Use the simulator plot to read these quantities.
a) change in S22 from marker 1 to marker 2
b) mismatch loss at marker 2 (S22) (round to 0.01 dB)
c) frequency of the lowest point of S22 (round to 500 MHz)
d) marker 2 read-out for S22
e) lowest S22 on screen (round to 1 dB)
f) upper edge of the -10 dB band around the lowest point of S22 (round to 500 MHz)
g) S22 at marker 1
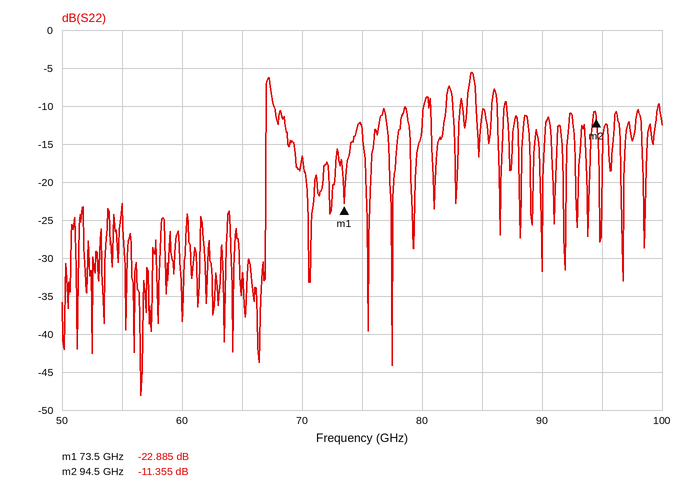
11.530 dB
0.33 dB
56.5 GHz
-11.355 dB
-48 dB
67.0 GHz
-22.885 dB
